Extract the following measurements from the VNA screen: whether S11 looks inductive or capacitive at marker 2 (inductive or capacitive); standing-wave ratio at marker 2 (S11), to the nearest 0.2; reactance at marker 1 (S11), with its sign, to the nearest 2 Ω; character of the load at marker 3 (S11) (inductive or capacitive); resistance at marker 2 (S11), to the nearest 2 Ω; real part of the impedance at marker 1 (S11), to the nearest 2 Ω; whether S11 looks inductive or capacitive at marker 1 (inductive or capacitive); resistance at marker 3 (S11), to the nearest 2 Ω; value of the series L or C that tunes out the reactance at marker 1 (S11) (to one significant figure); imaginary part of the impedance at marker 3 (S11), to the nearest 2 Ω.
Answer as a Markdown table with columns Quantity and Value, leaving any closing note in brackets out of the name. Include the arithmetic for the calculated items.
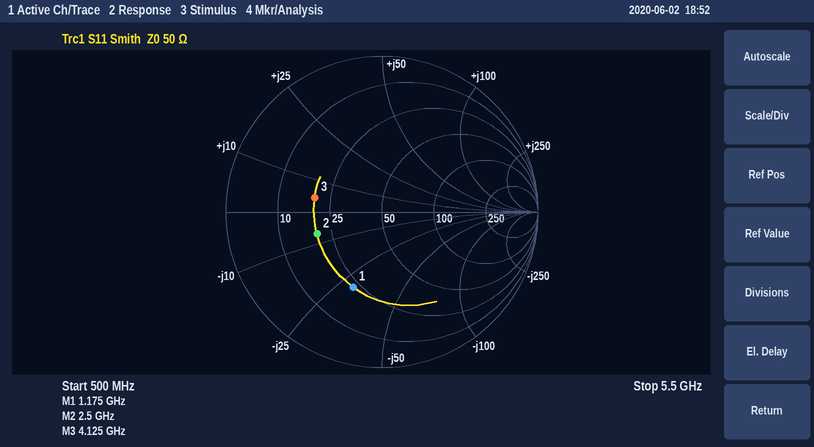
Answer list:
| Quantity | Value |
|---|---|
| whether S11 looks inductive or capacitive at marker 2 | capacitive |
| standing-wave ratio at marker 2 (S11), to the nearest 0.2 | 2.6 |
| reactance at marker 1 (S11), with its sign, to the nearest 2 Ω | -30 Ω |
| character of the load at marker 3 (S11) | inductive |
| resistance at marker 2 (S11), to the nearest 2 Ω | 20 Ω |
| real part of the impedance at marker 1 (S11), to the nearest 2 Ω | 22 Ω |
| whether S11 looks inductive or capacitive at marker 1 | capacitive |
| resistance at marker 3 (S11), to the nearest 2 Ω | 20 Ω |
| value of the series L or C that tunes out the reactance at marker 1 (S11) | L = 30 Ω/(2π × 1.175 GHz) ≈ 4 nH |
| imaginary part of the impedance at marker 3 (S11), to the nearest 2 Ω | +4 Ω |
